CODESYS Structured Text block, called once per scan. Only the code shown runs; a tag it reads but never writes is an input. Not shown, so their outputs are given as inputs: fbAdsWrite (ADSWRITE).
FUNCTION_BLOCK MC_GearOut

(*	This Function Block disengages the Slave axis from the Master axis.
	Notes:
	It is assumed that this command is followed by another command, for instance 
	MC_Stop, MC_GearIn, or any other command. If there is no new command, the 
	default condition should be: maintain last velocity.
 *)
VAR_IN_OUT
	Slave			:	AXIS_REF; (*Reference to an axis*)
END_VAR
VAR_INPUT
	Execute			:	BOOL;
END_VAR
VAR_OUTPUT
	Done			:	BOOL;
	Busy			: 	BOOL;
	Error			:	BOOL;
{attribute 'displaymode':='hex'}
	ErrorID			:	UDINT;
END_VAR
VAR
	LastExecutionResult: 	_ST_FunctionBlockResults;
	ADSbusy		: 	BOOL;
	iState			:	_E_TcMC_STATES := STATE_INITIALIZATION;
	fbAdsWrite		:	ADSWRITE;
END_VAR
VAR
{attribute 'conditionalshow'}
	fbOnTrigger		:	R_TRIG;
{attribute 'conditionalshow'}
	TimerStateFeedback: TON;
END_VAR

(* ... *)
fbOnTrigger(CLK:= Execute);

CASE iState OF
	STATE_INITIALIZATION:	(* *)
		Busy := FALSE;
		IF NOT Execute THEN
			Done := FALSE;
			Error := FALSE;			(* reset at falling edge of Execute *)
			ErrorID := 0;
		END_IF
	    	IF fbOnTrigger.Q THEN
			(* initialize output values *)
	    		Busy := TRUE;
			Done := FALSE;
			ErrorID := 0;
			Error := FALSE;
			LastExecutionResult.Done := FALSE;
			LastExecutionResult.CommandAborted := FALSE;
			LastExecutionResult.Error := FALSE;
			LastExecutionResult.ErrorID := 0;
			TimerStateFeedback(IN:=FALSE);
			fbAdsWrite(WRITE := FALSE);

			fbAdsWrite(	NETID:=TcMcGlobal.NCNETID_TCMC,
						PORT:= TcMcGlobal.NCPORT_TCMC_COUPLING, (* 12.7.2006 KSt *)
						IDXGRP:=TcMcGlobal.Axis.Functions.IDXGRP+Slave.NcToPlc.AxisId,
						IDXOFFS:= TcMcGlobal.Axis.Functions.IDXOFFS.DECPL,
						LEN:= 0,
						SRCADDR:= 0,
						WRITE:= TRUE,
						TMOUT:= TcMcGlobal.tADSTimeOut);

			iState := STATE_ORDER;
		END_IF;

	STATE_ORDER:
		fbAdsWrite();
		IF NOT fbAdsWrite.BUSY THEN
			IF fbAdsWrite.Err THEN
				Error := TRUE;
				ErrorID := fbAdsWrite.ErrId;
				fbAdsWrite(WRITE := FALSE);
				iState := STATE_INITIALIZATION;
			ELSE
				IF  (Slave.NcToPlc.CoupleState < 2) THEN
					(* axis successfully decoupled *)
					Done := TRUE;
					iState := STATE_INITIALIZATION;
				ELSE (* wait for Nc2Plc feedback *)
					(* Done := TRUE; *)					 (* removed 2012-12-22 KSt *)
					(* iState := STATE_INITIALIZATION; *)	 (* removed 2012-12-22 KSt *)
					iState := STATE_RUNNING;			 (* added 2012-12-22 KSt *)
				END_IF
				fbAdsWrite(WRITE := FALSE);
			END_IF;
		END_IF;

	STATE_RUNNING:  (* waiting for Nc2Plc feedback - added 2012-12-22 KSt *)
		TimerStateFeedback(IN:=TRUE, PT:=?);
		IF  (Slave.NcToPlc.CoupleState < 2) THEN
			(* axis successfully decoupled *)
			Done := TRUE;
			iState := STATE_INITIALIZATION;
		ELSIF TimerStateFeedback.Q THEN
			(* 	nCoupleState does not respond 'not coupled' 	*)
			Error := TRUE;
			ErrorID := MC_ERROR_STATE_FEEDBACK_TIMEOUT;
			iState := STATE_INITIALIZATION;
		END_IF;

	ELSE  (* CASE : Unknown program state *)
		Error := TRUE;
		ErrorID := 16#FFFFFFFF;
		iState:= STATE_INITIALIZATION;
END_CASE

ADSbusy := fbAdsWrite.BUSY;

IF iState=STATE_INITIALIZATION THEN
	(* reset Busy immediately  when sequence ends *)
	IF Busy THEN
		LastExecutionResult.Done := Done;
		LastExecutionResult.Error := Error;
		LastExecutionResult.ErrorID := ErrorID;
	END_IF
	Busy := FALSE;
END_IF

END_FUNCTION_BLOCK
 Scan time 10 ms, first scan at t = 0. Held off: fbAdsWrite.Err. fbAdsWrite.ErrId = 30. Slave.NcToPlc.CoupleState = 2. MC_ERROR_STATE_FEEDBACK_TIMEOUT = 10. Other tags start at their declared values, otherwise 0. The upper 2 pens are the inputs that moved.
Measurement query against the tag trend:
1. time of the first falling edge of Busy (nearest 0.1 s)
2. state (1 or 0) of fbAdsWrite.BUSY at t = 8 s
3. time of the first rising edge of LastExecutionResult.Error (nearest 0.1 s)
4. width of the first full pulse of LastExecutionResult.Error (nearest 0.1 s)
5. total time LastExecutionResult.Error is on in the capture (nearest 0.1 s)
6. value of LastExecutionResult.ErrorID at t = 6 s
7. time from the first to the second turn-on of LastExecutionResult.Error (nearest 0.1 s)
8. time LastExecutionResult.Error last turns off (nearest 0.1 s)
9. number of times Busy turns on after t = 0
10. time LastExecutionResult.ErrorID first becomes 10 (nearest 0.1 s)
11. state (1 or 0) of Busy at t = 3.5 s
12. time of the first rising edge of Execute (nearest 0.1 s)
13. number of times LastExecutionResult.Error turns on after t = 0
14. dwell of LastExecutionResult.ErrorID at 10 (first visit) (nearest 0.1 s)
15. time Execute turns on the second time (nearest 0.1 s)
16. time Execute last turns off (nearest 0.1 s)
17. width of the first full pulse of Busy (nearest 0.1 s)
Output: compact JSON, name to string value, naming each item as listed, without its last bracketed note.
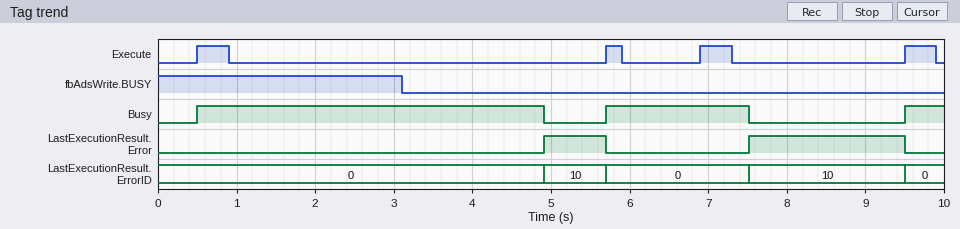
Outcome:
{"time of the first falling edge of Busy": "4.9 s", "state (1 or 0) of fbAdsWrite.BUSY at t = 8 s": "0", "time of the first rising edge of LastExecutionResult.Error": "4.9 s", "width of the first full pulse of LastExecutionResult.Error": "0.8 s", "total time LastExecutionResult.Error is on in the capture": "2.8 s", "value of LastExecutionResult.ErrorID at t = 6 s": "0", "time from the first to the second turn-on of LastExecutionResult.Error": "2.6 s", "time LastExecutionResult.Error last turns off": "9.5 s", "number of times Busy turns on after t = 0": "3", "time LastExecutionResult.ErrorID first becomes 10": "4.9 s", "state (1 or 0) of Busy at t = 3.5 s": "1", "time of the first rising edge of Execute": "0.5 s", "number of times LastExecutionResult.Error turns on after t = 0": "2", "dwell of LastExecutionResult.ErrorID at 10 (first visit)": "0.8 s", "time Execute turns on the second time": "5.7 s", "time Execute last turns off": "9.9 s", "width of the first full pulse of Busy": "4.4 s"}
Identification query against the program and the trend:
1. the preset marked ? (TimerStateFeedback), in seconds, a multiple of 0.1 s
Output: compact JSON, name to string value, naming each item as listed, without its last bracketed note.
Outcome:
{"the preset marked ? (TimerStateFeedback), in seconds, a multiple of 0.1 s": "1.8 s"}
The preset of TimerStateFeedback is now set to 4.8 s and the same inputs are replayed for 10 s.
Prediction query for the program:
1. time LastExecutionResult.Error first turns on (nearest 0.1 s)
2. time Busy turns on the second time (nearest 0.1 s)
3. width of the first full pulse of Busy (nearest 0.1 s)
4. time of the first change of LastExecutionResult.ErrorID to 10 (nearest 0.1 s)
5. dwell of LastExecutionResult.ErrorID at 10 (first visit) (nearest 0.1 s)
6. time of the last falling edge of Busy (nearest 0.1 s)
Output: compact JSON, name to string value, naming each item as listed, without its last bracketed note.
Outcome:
{"time LastExecutionResult.Error first turns on": "7.9 s", "time Busy turns on the second time": "9.5 s", "width of the first full pulse of Busy": "7.4 s", "time of the first change of LastExecutionResult.ErrorID to 10": "7.9 s", "dwell of LastExecutionResult.ErrorID at 10 (first visit)": "1.6 s", "time of the last falling edge of Busy": "7.9 s"}
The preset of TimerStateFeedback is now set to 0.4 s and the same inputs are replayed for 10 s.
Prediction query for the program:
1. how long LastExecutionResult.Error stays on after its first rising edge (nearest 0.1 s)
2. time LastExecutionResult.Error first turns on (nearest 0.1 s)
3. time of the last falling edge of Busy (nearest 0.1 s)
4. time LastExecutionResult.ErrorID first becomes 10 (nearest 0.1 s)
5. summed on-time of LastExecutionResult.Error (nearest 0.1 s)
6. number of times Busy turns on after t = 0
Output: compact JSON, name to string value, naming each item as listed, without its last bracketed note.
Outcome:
{"how long LastExecutionResult.Error stays on after its first rising edge": "2.2 s", "time LastExecutionResult.Error first turns on": "3.5 s", "time of the last falling edge of Busy": "9.9 s", "time LastExecutionResult.ErrorID first becomes 10": "3.5 s", "summed on-time of LastExecutionResult.Error": "5.2 s", "number of times Busy turns on after t = 0": "4"}
